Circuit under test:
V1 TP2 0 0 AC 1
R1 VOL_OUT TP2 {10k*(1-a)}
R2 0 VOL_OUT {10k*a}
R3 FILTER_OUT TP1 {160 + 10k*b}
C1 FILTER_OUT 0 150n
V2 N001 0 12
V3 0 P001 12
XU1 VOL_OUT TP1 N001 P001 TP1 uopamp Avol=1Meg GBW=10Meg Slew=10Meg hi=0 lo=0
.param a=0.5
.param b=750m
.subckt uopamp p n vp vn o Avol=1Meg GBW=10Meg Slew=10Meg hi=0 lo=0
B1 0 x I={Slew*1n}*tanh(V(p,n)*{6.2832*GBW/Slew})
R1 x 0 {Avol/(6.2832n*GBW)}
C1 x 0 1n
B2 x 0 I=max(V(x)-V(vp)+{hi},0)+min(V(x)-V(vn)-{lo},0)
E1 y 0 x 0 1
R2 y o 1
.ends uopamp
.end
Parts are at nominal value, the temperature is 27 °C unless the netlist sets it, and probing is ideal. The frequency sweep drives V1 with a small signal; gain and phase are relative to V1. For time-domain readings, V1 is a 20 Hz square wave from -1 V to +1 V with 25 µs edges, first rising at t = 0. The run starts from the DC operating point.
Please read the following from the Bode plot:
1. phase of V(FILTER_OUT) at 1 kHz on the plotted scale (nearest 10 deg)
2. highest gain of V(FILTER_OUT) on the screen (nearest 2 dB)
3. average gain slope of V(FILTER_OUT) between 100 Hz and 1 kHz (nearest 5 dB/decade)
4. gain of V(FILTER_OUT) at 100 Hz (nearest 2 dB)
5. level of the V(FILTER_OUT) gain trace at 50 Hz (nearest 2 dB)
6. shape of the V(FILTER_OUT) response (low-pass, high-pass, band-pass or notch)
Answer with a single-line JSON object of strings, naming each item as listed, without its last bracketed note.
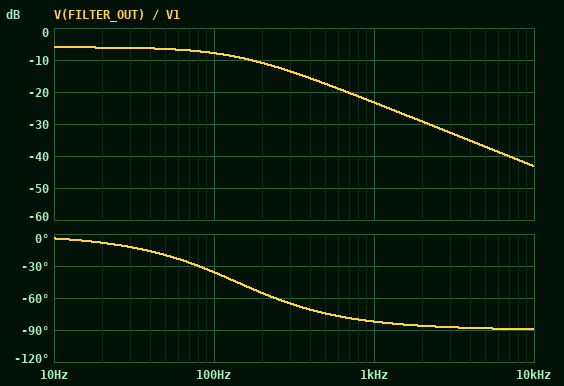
{"phase of V(FILTER_OUT) at 1 kHz on the plotted scale": "-80 deg", "highest gain of V(FILTER_OUT) on the screen": "-6 dB", "average gain slope of V(FILTER_OUT) between 100 Hz and 1 kHz": "-15 dB/decade", "gain of V(FILTER_OUT) at 100 Hz": "-8 dB", "level of the V(FILTER_OUT) gain trace at 50 Hz": "-6 dB", "shape of the V(FILTER_OUT) response": "low-pass"}
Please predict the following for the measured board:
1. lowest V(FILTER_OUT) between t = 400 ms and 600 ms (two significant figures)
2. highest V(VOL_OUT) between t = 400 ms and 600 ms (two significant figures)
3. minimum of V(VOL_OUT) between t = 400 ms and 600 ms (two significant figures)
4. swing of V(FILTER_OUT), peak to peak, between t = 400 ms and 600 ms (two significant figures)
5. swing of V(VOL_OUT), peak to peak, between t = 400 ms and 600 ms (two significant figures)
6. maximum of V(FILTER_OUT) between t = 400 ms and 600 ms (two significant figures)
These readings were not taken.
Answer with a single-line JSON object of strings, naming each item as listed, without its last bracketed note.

{"lowest V(FILTER_OUT) between t = 400 ms and 600 ms": "-500 mV", "highest V(VOL_OUT) between t = 400 ms and 600 ms": "500 mV", "minimum of V(VOL_OUT) between t = 400 ms and 600 ms": "-500 mV", "swing of V(FILTER_OUT), peak to peak, between t = 400 ms and 600 ms": "1.0 V", "swing of V(VOL_OUT), peak to peak, between t = 400 ms and 600 ms": "1.0 V", "maximum of V(FILTER_OUT) between t = 400 ms and 600 ms": "500 mV"}
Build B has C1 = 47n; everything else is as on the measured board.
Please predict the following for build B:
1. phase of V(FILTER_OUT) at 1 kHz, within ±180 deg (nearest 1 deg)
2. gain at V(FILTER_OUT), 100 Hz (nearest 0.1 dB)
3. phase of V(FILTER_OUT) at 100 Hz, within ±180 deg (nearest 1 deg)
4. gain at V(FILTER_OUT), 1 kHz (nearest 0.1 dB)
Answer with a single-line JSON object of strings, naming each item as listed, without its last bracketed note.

{"phase of V(FILTER_OUT) at 1 kHz, within ±180 deg": "-66 deg", "gain at V(FILTER_OUT), 100 Hz": "-6.2 dB", "phase of V(FILTER_OUT) at 100 Hz, within ±180 deg": "-13 deg", "gain at V(FILTER_OUT), 1 kHz": "-13.9 dB"}
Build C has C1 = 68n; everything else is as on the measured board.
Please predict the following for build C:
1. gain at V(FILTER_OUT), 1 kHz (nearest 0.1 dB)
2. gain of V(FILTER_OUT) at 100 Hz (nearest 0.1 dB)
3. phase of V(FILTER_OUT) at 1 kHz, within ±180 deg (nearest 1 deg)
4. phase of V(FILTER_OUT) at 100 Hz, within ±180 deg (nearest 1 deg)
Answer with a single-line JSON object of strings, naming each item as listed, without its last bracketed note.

{"gain at V(FILTER_OUT), 1 kHz": "-16.7 dB", "gain of V(FILTER_OUT) at 100 Hz": "-6.5 dB", "phase of V(FILTER_OUT) at 1 kHz, within ±180 deg": "-73 deg", "phase of V(FILTER_OUT) at 100 Hz, within ±180 deg": "-18 deg"}
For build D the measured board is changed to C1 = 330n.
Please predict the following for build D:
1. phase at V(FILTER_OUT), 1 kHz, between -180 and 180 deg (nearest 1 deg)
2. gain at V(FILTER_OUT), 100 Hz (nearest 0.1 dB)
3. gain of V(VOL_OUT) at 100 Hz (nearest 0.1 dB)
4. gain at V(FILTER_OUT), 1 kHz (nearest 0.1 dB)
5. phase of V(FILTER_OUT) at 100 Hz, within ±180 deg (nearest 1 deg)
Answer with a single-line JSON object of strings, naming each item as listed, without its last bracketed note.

{"phase at V(FILTER_OUT), 1 kHz, between -180 and 180 deg": "-86 deg", "gain at V(FILTER_OUT), 100 Hz": "-11.5 dB", "gain of V(VOL_OUT) at 100 Hz": "-6.0 dB", "gain at V(FILTER_OUT), 1 kHz": "-30.1 dB", "phase of V(FILTER_OUT) at 100 Hz, within ±180 deg": "-58 deg"}
